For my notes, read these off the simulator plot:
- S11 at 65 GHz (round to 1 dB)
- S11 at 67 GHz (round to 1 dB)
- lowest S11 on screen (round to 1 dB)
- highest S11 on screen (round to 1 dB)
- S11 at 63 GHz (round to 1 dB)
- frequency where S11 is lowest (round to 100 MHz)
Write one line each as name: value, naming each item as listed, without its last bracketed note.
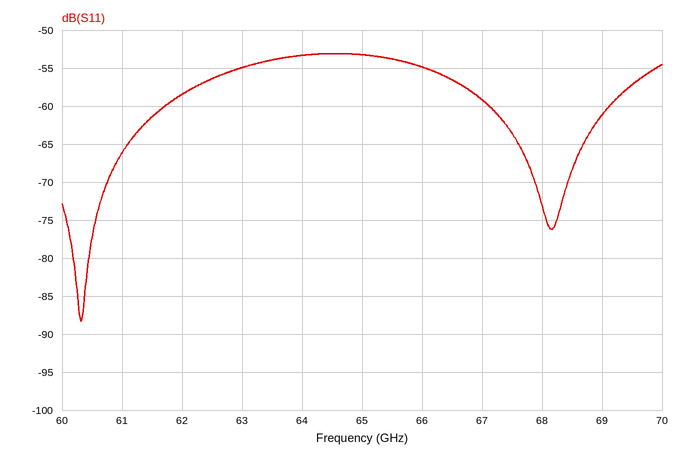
S11 at 65 GHz: -53 dB
S11 at 67 GHz: -59 dB
lowest S11 on screen: -88 dB
highest S11 on screen: -53 dB
S11 at 63 GHz: -55 dB
frequency where S11 is lowest: 60.3 GHz
